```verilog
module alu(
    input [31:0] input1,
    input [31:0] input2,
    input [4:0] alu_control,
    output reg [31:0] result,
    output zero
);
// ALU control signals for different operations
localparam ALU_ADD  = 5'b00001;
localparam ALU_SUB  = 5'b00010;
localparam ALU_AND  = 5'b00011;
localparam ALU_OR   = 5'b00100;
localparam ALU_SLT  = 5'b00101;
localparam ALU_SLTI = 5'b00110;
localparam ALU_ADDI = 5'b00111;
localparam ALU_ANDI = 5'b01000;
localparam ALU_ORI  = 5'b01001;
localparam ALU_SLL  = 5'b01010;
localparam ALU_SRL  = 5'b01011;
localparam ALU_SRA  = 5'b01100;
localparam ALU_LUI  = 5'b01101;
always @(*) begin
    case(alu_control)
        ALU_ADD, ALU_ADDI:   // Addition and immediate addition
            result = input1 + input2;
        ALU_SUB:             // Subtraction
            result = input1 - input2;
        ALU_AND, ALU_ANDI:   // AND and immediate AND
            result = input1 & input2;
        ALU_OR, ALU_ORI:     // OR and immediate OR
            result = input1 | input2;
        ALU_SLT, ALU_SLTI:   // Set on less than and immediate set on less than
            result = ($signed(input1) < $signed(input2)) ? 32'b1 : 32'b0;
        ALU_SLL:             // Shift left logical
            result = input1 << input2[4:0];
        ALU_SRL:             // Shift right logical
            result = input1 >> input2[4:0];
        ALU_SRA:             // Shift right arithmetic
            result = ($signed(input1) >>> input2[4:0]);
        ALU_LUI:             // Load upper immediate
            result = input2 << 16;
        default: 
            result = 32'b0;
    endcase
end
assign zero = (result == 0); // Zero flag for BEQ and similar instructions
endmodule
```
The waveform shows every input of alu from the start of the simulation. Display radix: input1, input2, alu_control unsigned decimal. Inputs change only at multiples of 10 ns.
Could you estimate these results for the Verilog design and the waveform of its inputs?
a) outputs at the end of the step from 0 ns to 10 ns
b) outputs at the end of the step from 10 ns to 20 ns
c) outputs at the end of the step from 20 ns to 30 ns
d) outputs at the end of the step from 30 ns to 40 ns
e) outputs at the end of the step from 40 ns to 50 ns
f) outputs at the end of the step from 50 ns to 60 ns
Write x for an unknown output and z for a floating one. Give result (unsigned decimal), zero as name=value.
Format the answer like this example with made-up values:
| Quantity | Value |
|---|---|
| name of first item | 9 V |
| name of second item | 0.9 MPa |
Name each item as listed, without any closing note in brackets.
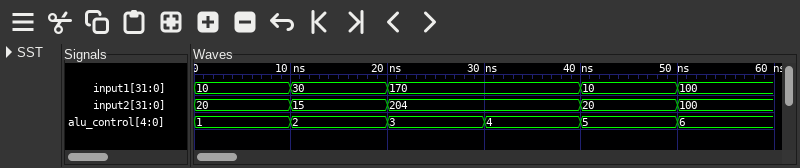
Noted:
| Quantity | Value |
|---|---|
| outputs at the end of the step from 0 ns to 10 ns | result=30, zero=0 |
| outputs at the end of the step from 10 ns to 20 ns | result=15, zero=0 |
| outputs at the end of the step from 20 ns to 30 ns | result=136, zero=0 |
| outputs at the end of the step from 30 ns to 40 ns | result=238, zero=0 |
| outputs at the end of the step from 40 ns to 50 ns | result=1, zero=0 |
| outputs at the end of the step from 50 ns to 60 ns | result=0, zero=1 |
